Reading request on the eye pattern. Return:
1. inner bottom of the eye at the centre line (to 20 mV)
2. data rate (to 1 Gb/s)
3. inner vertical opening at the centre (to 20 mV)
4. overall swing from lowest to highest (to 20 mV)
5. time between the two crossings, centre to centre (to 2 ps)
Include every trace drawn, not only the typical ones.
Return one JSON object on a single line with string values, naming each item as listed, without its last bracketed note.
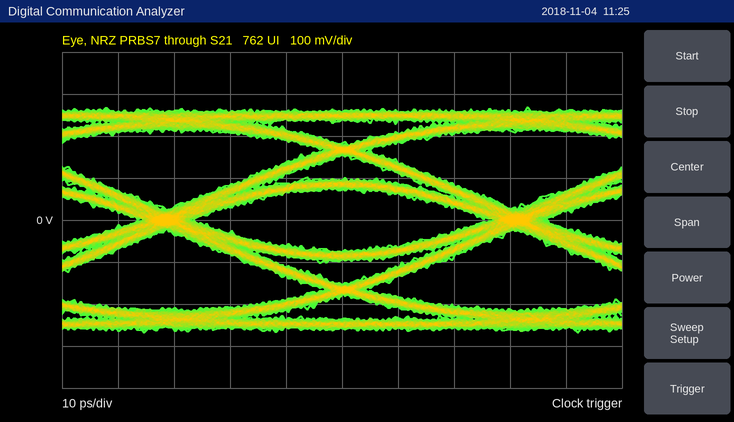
{"inner bottom of the eye at the centre line": "-80 mV", "data rate": "16 Gb/s", "inner vertical opening at the centre": "140 mV", "overall swing from lowest to highest": "540 mV", "time between the two crossings, centre to centre": "62 ps"}
